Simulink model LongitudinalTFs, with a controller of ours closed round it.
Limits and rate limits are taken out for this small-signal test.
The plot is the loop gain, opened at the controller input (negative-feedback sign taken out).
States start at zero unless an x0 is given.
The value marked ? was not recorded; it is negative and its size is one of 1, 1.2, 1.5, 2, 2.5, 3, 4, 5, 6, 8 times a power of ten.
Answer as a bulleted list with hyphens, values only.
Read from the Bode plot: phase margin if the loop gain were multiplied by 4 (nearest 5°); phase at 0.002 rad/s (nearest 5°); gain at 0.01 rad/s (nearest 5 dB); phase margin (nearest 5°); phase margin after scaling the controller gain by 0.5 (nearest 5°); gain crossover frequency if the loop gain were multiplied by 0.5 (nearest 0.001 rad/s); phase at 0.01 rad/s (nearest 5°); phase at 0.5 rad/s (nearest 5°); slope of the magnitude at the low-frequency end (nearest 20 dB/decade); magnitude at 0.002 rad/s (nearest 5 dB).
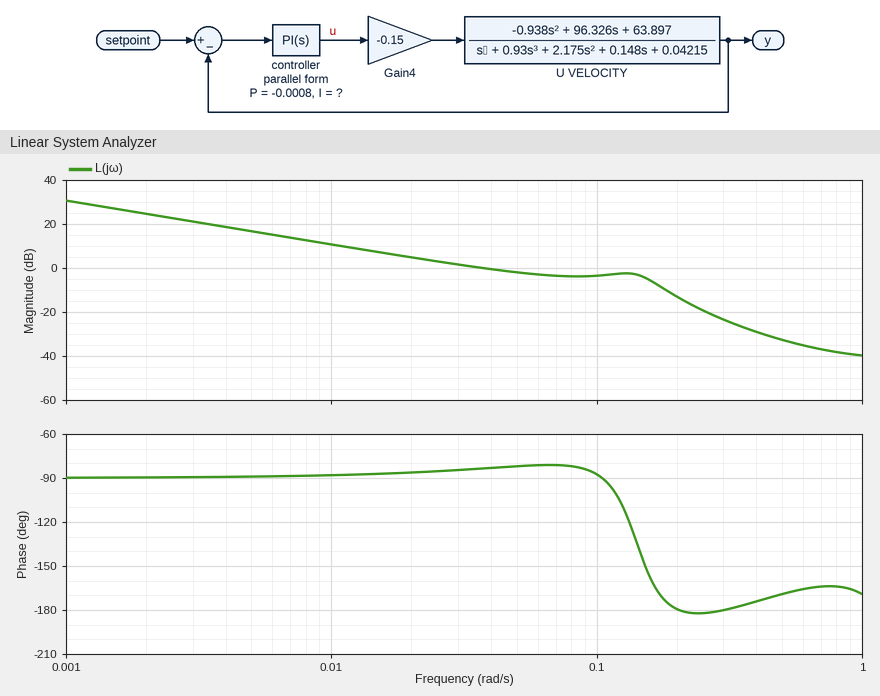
- 0°
- -90°
- 10 dB
- 95°
- 95°
- 0.017 rad/s
- -90°
- -170°
- -20 dB/decade
- 25 dB
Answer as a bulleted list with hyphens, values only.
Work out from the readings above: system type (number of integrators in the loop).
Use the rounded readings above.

- 1
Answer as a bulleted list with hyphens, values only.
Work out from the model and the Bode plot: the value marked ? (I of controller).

- -0.00015
